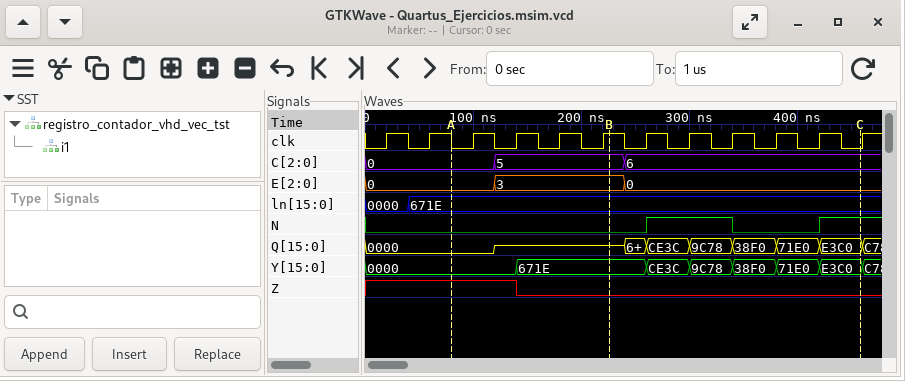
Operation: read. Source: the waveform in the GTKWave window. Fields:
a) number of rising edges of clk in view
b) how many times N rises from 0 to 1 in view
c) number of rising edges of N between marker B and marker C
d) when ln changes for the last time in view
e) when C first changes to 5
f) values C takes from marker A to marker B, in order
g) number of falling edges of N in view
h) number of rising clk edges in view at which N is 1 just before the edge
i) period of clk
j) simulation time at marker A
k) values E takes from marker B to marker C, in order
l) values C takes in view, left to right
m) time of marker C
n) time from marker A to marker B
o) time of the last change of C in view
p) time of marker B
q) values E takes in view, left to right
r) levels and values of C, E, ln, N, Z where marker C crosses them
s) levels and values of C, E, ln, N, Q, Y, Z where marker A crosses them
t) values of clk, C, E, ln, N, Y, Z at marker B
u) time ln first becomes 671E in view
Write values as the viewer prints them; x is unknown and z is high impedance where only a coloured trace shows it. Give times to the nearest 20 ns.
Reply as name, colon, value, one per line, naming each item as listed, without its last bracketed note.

number of rising edges of clk in view: 12
how many times N rises from 0 to 1 in view: 2
number of rising edges of N between marker B and marker C: 2
when ln changes for the last time in view: 40 ns
when C first changes to 5: 120 ns
values C takes from marker A to marker B, in order: 0, 5
number of falling edges of N in view: 1
number of rising clk edges in view at which N is 1 just before the edge: 3
period of clk: 40 ns
simulation time at marker A: 80 ns
values E takes from marker B to marker C, in order: 3, 0
values C takes in view, left to right: 0, 5, 6
time of marker C: 460 ns
time from marker A to marker B: 140 ns
time of the last change of C in view: 240 ns
time of marker B: 220 ns
values E takes in view, left to right: 0, 3, 0
levels and values of C, E, ln, N, Z where marker C crosses them: C=6, E=0, ln=671E, N=1, Z=0
levels and values of C, E, ln, N, Q, Y, Z where marker A crosses them: C=0, E=0, ln=671E, N=0, Q=0000, Y=0000, Z=1
values of clk, C, E, ln, N, Y, Z at marker B: clk=1, C=5, E=3, ln=671E, N=0, Y=671E, Z=0
time ln first becomes 671E in view: 40 ns
